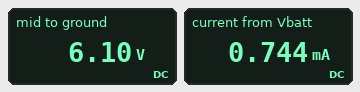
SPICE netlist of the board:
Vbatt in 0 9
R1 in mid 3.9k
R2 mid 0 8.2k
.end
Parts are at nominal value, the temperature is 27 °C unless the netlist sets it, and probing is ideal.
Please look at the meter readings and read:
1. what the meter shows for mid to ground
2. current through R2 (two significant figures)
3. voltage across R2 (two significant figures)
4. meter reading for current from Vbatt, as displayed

6.10 V
740 µA
6.1 V
0.744 mA
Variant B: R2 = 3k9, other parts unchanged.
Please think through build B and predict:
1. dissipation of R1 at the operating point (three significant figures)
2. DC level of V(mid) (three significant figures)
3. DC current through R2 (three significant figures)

5.19 mW
4.50 V
1.15 mA
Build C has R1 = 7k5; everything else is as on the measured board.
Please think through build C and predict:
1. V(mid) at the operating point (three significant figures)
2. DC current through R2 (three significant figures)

4.70 V
573 µA
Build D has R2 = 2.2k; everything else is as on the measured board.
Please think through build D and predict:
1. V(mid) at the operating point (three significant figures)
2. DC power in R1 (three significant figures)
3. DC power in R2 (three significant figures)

3.25 V
8.49 mW
4.79 mW
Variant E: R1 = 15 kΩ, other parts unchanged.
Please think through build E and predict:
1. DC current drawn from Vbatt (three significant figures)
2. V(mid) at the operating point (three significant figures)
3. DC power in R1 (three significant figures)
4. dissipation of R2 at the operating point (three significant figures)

388 µA
3.18 V
2.26 mW
1.23 mW
